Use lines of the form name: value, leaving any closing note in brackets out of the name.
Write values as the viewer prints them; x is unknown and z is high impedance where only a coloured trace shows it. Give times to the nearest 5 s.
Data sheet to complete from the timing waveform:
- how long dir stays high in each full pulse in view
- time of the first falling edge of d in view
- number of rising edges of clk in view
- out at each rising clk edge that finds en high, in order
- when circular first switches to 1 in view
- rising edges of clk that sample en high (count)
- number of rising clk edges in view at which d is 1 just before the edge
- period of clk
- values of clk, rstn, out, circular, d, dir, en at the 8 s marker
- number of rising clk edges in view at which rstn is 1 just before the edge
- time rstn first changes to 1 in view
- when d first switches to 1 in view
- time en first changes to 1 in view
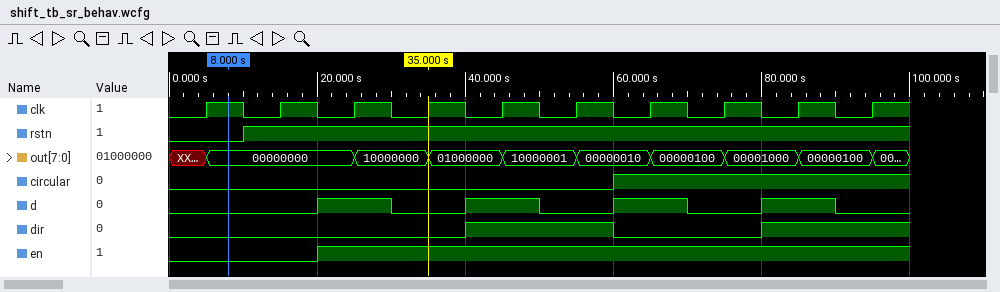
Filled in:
how long dir stays high in each full pulse in view: 20 s
time of the first falling edge of d in view: 30 s
number of rising edges of clk in view: 10
out at each rising clk edge that finds en high, in order: 00000000, 10000000, 01000000, 10000001, 00000010, 00000100, 00001000, 00000100
when circular first switches to 1 in view: 60 s
rising edges of clk that sample en high: 8
number of rising clk edges in view at which d is 1 just before the edge: 4
period of clk: 10 s
values of clk, rstn, out, circular, d, dir, en at the 8 s marker: clk=1, rstn=0, out=00000000, circular=0, d=0, dir=0, en=0
number of rising clk edges in view at which rstn is 1 just before the edge: 9
time rstn first changes to 1 in view: 10 s
when d first switches to 1 in view: 20 s
time en first changes to 1 in view: 20 s
